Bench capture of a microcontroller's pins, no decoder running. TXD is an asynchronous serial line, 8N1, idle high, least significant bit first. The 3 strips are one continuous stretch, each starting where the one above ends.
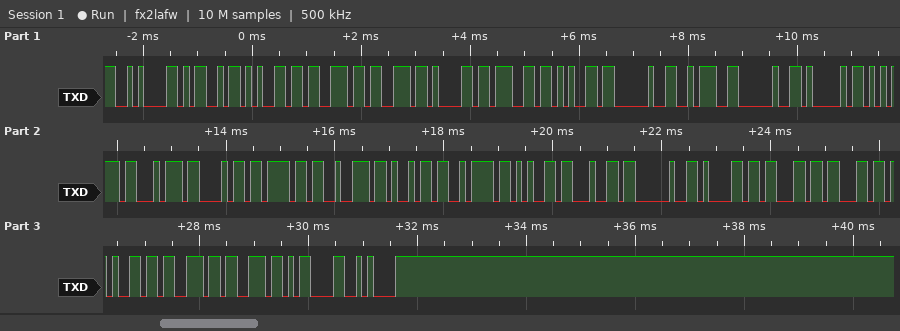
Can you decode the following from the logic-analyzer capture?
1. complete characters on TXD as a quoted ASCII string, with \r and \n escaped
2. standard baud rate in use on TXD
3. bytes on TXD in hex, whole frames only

"\nMessage : Authorized access\r\n"
9600 baud
0x0A 0x4D 0x65 0x73 0x73 0x61 0x67 0x65 0x20 0x3A 0x20 0x41 0x75 0x74 0x68 0x6F 0x72 0x69 0x7A 0x65 0x64 0x20 0x61 0x63 0x63 0x65 0x73 0x73 0x0D 0x0A
